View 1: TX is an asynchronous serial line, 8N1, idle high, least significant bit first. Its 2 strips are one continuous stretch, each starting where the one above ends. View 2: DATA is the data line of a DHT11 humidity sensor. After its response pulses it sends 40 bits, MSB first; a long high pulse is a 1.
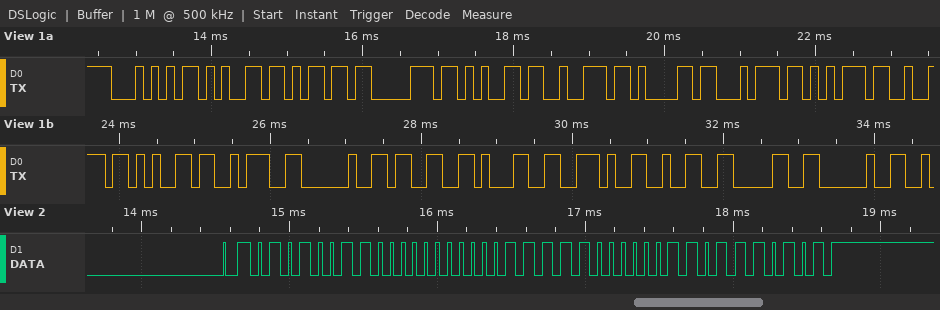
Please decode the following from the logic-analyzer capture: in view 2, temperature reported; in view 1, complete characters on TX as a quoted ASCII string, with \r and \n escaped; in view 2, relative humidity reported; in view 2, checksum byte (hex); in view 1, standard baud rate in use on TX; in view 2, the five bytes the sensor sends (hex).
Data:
31.3 °C
"Temperature: 31.20 "
83 %
0x75
9600 baud
53 00 1F 03 75
